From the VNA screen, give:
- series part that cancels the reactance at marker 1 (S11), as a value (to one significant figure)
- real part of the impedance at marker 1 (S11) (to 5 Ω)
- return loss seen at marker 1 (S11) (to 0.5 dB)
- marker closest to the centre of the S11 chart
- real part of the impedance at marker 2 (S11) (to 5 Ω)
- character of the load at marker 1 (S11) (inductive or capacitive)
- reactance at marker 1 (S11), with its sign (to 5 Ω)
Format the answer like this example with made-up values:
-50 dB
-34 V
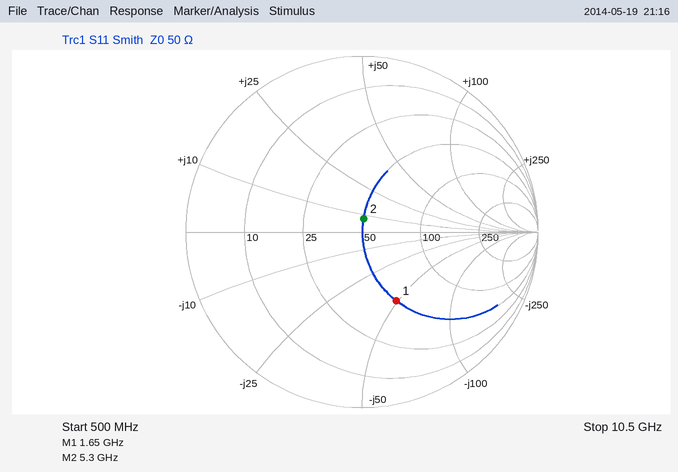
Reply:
5 nH
50 Ω
7.0 dB
marker 2
50 Ω
capacitive
-50 Ω
